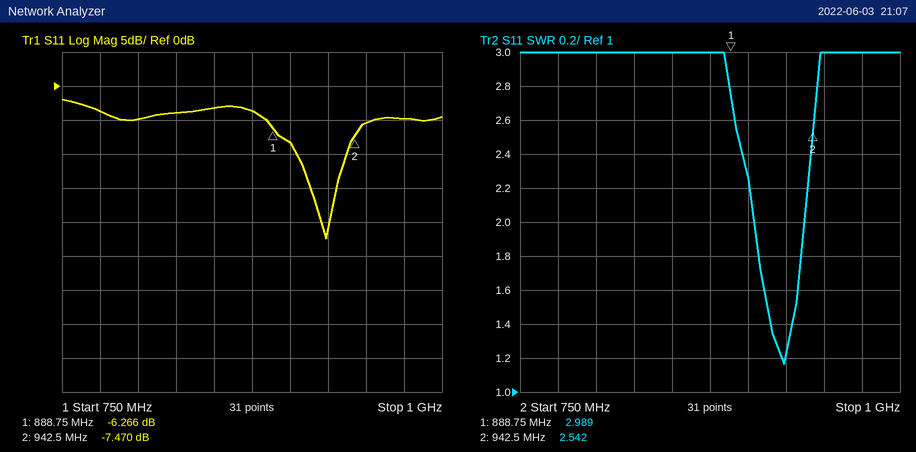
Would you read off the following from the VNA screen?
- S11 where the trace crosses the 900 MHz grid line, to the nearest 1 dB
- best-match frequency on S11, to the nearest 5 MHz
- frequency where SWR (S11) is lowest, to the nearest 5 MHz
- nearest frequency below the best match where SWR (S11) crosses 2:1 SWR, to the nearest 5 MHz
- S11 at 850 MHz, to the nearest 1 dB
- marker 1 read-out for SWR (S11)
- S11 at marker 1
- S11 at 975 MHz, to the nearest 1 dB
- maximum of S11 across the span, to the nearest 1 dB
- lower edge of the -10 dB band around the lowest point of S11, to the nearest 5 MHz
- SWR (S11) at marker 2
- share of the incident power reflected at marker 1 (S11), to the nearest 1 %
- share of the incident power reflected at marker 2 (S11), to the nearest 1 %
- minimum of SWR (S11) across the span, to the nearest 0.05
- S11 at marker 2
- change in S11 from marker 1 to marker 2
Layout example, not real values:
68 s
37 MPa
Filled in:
-8 dB
925 MHz
925 MHz
905 MHz
-3 dB
2.989
-6.266 dB
-5 dB
-2 dB
905 MHz
2.542
24 %
18 %
1.15
-7.470 dB
-1.204 dB
